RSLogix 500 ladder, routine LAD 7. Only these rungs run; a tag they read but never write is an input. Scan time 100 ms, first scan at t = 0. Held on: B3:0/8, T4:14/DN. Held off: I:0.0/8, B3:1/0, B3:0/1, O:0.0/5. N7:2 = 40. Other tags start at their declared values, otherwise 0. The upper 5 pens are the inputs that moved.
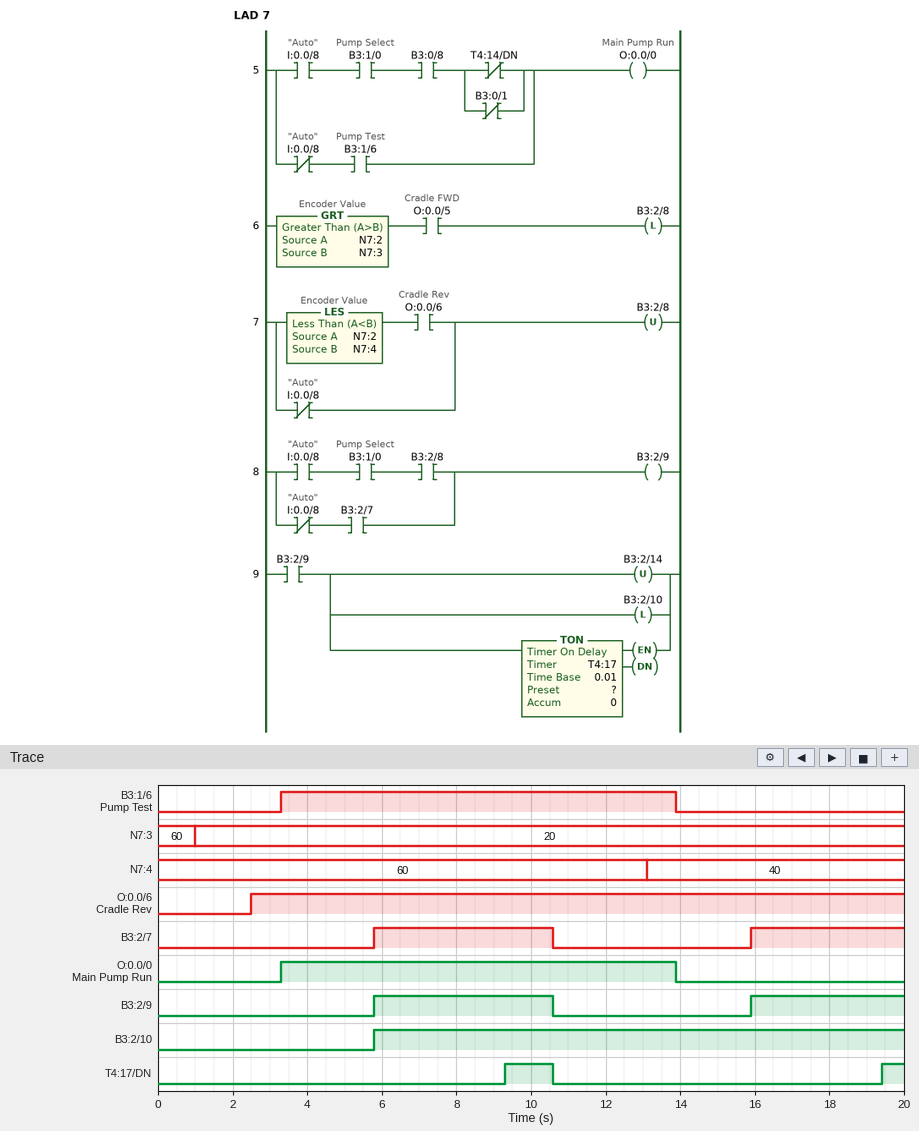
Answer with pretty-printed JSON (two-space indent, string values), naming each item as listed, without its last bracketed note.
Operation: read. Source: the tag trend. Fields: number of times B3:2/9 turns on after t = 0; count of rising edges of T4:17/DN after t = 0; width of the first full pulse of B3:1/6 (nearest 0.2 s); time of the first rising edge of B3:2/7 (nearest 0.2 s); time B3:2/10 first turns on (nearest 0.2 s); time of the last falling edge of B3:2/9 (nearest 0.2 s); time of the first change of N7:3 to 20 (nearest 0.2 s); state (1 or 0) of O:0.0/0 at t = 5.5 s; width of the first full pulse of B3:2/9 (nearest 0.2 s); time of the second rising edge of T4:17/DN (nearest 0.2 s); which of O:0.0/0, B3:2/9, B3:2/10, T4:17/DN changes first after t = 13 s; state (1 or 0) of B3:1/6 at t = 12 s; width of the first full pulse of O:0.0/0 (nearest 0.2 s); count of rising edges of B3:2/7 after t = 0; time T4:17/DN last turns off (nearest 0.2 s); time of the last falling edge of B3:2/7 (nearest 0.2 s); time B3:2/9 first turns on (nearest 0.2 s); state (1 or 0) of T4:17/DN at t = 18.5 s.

{
  "number of times B3:2/9 turns on after t = 0": "2",
  "count of rising edges of T4:17/DN after t = 0": "2",
  "width of the first full pulse of B3:1/6": "10.6 s",
  "time of the first rising edge of B3:2/7": "5.8 s",
  "time B3:2/10 first turns on": "5.8 s",
  "time of the last falling edge of B3:2/9": "10.6 s",
  "time of the first change of N7:3 to 20": "1.0 s",
  "state (1 or 0) of O:0.0/0 at t = 5.5 s": "1",
  "width of the first full pulse of B3:2/9": "4.8 s",
  "time of the second rising edge of T4:17/DN": "19.4 s",
  "which of O:0.0/0, B3:2/9, B3:2/10, T4:17/DN changes first after t = 13 s": "O:0.0/0",
  "state (1 or 0) of B3:1/6 at t = 12 s": "1",
  "width of the first full pulse of O:0.0/0": "10.6 s",
  "count of rising edges of B3:2/7 after t = 0": "2",
  "time T4:17/DN last turns off": "10.6 s",
  "time of the last falling edge of B3:2/7": "10.6 s",
  "time B3:2/9 first turns on": "5.8 s",
  "state (1 or 0) of T4:17/DN at t = 18.5 s": "0"
}
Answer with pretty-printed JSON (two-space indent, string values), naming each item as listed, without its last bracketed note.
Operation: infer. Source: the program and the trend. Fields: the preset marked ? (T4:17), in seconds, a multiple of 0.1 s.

{
  "the preset marked ? (T4:17), in seconds, a multiple of 0.1 s": "3.5 s"
}
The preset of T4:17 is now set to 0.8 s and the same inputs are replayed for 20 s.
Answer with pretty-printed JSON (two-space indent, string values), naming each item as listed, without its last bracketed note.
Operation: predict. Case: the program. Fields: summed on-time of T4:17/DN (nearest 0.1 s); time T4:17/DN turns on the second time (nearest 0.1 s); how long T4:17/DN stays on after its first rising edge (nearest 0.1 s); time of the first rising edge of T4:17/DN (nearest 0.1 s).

{
  "summed on-time of T4:17/DN": "7.3 s",
  "time T4:17/DN turns on the second time": "16.7 s",
  "how long T4:17/DN stays on after its first rising edge": "4.0 s",
  "time of the first rising edge of T4:17/DN": "6.6 s"
}
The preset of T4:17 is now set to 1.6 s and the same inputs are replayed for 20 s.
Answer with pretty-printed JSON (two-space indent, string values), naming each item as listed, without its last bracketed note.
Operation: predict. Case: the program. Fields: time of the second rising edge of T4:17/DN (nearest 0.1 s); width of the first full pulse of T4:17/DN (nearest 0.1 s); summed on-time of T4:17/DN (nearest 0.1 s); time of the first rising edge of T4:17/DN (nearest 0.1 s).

{
  "time of the second rising edge of T4:17/DN": "17.5 s",
  "width of the first full pulse of T4:17/DN": "3.2 s",
  "summed on-time of T4:17/DN": "5.7 s",
  "time of the first rising edge of T4:17/DN": "7.4 s"
}
